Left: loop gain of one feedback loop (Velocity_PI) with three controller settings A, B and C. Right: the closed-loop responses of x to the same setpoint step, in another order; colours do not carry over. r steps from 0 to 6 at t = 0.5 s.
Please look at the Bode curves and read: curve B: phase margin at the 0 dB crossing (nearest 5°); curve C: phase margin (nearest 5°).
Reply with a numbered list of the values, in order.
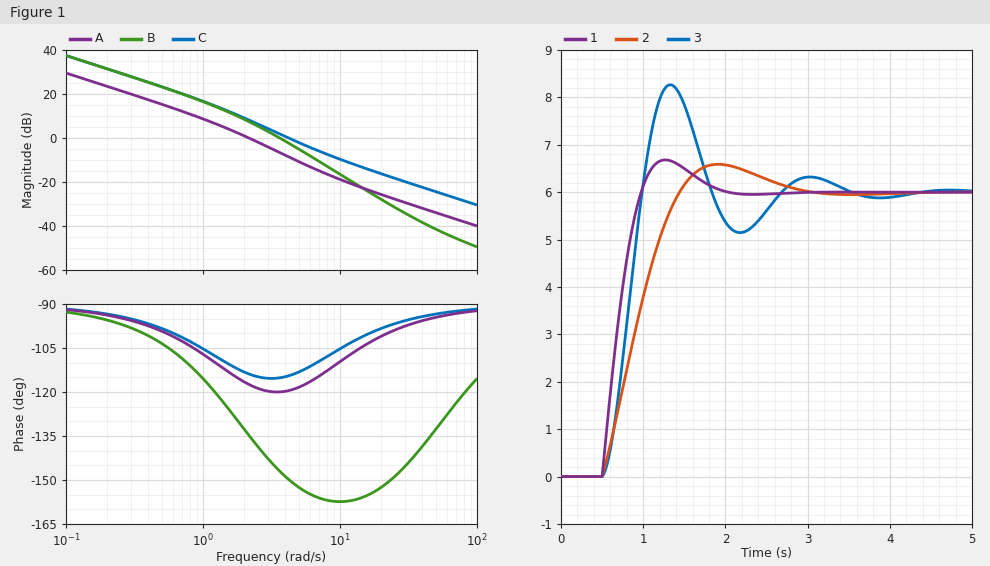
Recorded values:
1. 35°
2. 65°
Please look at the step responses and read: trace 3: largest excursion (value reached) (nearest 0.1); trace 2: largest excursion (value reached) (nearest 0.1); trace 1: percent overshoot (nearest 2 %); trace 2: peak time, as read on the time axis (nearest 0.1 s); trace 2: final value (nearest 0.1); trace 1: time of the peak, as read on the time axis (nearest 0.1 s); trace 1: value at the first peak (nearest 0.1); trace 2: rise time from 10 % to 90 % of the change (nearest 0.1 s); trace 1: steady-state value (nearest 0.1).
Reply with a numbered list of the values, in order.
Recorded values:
1. 8.3
2. 6.6
3. 12 %
4. 1.9 s
5. 6.0
6. 1.3 s
7. 6.7
8. 0.7 s
9. 6.0
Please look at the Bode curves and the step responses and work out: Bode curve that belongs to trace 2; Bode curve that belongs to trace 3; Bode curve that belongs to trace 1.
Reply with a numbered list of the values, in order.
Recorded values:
1. A
2. B
3. C
